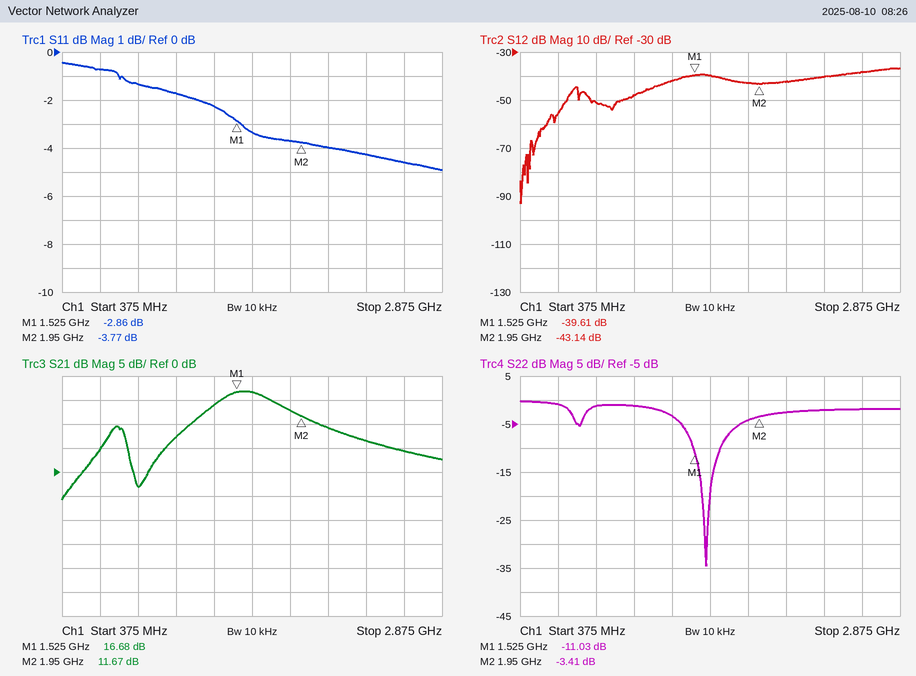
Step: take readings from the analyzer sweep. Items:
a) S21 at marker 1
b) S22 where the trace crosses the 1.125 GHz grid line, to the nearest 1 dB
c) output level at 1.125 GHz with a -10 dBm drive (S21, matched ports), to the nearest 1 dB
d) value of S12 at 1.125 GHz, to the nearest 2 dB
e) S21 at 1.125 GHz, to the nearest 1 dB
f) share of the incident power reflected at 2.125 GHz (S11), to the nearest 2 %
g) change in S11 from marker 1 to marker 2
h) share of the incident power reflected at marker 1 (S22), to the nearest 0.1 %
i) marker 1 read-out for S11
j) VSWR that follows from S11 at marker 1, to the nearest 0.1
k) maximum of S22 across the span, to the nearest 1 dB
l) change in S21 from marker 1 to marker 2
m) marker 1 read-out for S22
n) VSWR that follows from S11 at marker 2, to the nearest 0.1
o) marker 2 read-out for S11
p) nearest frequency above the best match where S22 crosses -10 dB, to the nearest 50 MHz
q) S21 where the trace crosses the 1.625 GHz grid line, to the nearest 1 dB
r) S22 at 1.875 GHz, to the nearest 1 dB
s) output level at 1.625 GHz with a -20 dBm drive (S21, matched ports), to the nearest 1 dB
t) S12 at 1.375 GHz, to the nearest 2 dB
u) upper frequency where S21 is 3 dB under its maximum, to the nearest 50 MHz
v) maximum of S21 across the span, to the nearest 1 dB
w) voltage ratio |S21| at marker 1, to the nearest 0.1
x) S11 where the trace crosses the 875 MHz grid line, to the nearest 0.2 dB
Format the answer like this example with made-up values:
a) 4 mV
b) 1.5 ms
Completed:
a) 16.68 dB
b) -1 dB
c) -3 dBm
d) -48 dB
e) 7 dB
f) 40 %
g) -0.91 dB
h) 7.9 %
i) -2.86 dB
j) 6.1
k) 0 dB
l) -5.01 dB
m) -11.03 dB
n) 4.7
o) -3.77 dB
p) 1.70 GHz
q) 17 dB
r) -4 dB
s) -3 dBm
t) -42 dB
u) 1.80 GHz
v) 17 dB
w) 6.8
x) -1.4 dB
